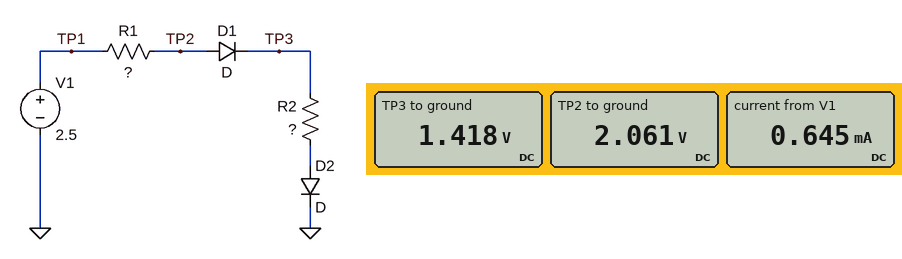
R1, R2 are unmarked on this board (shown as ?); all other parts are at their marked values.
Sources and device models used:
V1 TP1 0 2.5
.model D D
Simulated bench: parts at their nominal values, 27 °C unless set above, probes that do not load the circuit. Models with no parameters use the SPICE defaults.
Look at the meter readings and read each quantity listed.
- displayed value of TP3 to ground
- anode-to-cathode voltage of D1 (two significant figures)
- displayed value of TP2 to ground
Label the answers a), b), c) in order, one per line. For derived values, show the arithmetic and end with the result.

a) 1.418 V
b) 2.061 V - 1.418 V = 640 mV
c) 2.061 V
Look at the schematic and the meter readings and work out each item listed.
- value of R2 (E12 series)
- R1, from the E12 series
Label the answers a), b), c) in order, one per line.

a) 1.2 kΩ
b) 680 Ω
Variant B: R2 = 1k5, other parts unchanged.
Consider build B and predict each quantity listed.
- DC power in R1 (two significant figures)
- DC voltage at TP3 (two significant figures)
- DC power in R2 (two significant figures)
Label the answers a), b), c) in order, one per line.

a) 210 µW
b) 1.5 V
c) 470 µW
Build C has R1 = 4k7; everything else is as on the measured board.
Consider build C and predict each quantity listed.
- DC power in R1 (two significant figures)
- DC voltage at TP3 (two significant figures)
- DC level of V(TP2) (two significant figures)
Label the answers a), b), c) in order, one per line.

a) 220 µW
b) 870 mV
c) 1.5 V
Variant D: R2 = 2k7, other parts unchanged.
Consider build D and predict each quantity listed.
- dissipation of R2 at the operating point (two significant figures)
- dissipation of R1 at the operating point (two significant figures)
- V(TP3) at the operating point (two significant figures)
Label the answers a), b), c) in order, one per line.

a) 360 µW
b) 92 µW
c) 1.6 V
